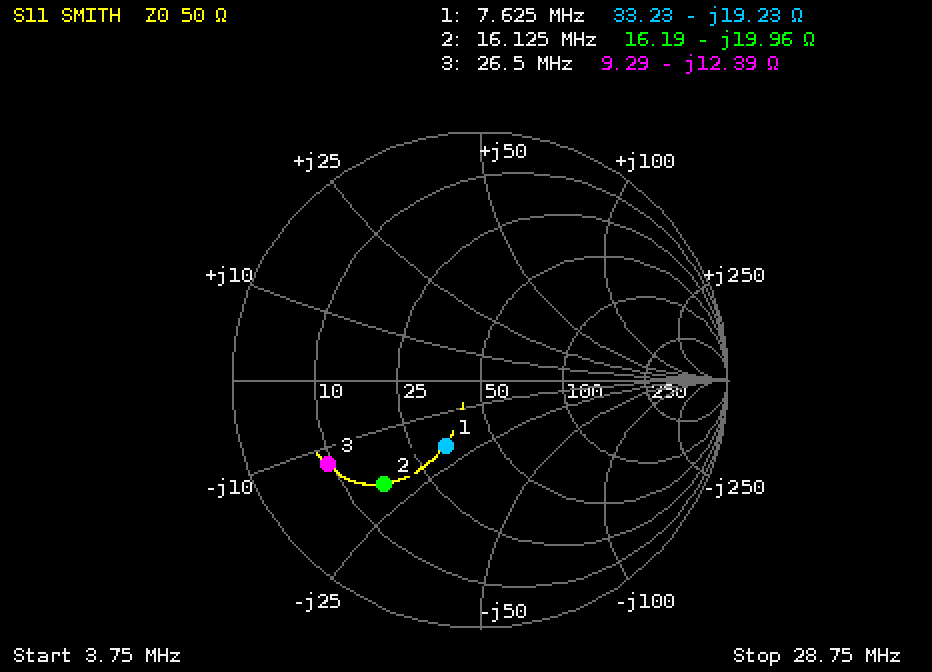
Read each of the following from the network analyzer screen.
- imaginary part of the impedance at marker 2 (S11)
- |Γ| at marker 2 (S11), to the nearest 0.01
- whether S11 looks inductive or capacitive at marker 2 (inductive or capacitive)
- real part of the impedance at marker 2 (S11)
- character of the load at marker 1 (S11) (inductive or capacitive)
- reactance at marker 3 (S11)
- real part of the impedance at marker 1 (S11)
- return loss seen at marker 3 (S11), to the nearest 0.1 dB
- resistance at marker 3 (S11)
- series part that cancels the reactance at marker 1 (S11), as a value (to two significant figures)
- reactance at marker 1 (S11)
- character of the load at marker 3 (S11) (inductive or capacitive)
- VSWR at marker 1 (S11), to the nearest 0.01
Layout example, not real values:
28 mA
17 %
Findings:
-19.96 Ω
0.57
capacitive
16.19 Ω
capacitive
-12.39 Ω
33.23 Ω
3.1 dB
9.29 Ω
400 nH
-19.23 Ω
capacitive
1.85
